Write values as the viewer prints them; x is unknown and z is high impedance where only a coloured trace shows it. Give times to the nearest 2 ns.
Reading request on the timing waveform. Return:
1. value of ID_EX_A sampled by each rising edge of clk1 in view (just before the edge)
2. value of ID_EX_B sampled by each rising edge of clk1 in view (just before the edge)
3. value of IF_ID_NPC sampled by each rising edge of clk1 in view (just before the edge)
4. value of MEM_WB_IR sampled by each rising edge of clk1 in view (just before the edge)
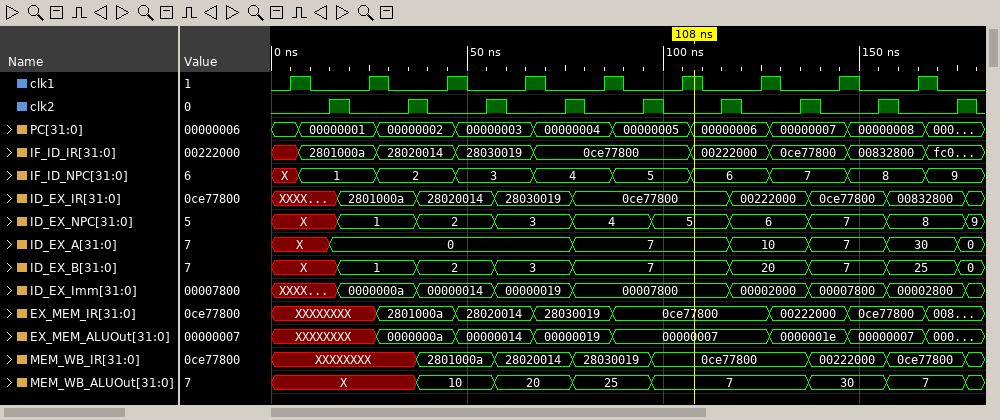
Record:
X, 0, 0, 0, 7, 7, 10, 7, 30
X, 1, 2, 3, 7, 7, 20, 7, 25
X, 1, 2, 3, 4, 5, 6, 7, 8
XXXXXXXX, XXXXXXXX, 2801000a, 28020014, 28030019, 0ce77800, 0ce77800, 00222000, 0ce77800
